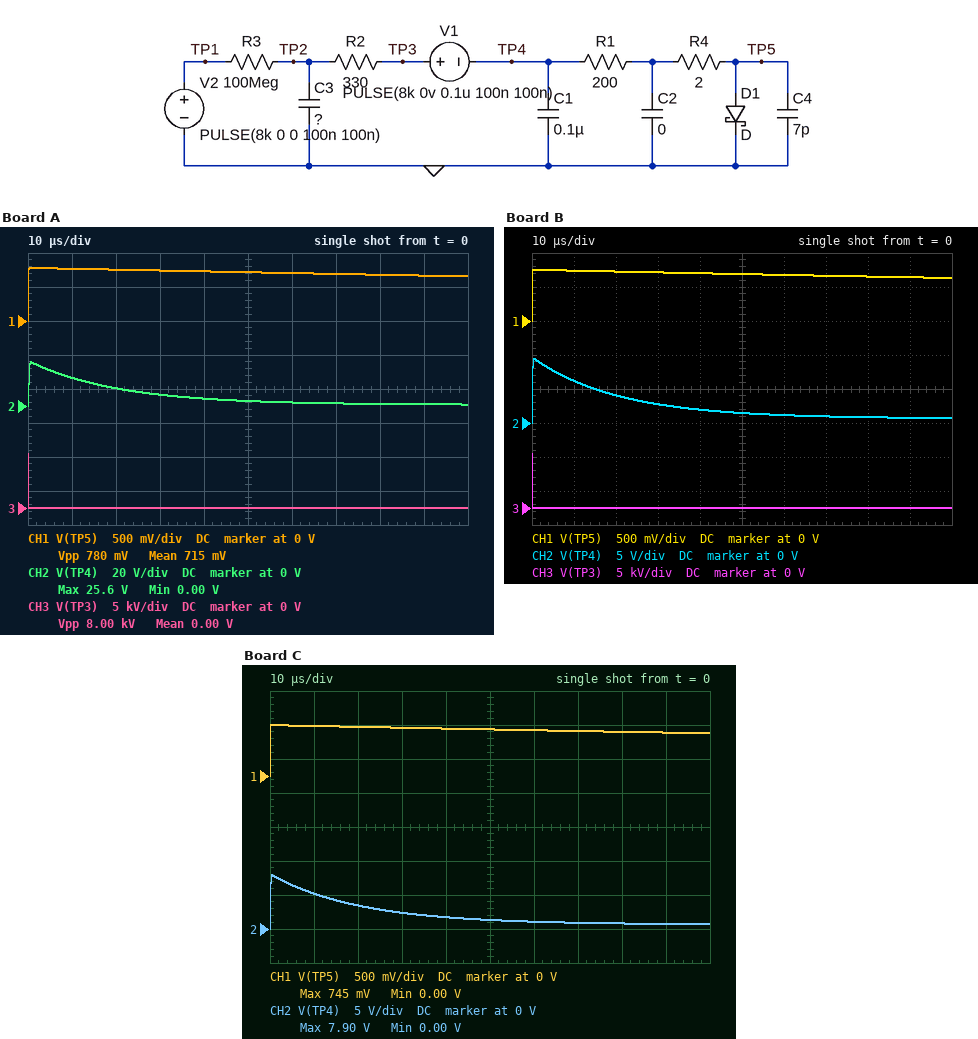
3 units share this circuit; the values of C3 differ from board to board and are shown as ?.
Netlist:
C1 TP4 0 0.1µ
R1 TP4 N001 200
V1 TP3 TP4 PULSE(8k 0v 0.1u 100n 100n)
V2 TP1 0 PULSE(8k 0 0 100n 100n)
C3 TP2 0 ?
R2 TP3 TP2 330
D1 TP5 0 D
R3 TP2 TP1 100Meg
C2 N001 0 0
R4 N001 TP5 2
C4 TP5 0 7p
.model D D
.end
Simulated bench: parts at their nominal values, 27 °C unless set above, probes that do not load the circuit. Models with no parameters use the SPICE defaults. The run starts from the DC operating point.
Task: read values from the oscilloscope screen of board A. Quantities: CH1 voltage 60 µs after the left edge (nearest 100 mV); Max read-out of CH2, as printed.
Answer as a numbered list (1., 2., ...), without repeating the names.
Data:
1. 700 mV
2. 25.6 V
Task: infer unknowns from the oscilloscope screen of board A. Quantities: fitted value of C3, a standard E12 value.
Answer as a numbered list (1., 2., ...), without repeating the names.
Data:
1. 330 pF
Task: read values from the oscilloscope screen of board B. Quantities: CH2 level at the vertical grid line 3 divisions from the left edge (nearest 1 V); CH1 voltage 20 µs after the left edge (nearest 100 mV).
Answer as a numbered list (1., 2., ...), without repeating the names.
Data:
1. 3 V
2. 700 mV
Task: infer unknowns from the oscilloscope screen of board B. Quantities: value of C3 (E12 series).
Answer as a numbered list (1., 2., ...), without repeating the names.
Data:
1. 120 pF
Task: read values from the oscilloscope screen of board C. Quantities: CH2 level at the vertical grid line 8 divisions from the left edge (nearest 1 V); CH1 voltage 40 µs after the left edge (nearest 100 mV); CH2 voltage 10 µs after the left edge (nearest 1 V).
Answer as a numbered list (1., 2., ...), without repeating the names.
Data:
1. 1 V
2. 700 mV
3. 5 V
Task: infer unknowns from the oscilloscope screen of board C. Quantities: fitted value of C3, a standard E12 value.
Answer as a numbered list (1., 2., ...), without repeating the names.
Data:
1. 100 pF
